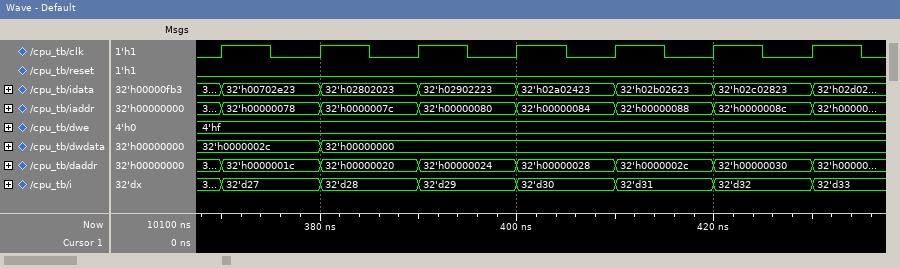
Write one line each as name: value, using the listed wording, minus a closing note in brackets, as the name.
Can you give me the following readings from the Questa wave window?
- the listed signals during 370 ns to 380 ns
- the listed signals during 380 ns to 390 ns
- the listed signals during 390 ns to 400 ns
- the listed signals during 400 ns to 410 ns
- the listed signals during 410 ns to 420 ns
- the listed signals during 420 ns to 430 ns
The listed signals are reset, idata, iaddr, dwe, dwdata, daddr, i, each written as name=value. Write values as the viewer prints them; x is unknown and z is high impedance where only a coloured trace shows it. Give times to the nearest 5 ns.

the listed signals during 370 ns to 380 ns: reset=0, idata=32'h00702e23, iaddr=32'h00000078, dwe=4'hf, dwdata=32'h0000002c, daddr=32'h0000001c, i=32'd27
the listed signals during 380 ns to 390 ns: reset=0, idata=32'h02802023, iaddr=32'h0000007c, dwe=4'hf, dwdata=32'h00000000, daddr=32'h00000020, i=32'd28
the listed signals during 390 ns to 400 ns: reset=0, idata=32'h02902223, iaddr=32'h00000080, dwe=4'hf, dwdata=32'h00000000, daddr=32'h00000024, i=32'd29
the listed signals during 400 ns to 410 ns: reset=0, idata=32'h02a02423, iaddr=32'h00000084, dwe=4'hf, dwdata=32'h00000000, daddr=32'h00000028, i=32'd30
the listed signals during 410 ns to 420 ns: reset=0, idata=32'h02b02623, iaddr=32'h00000088, dwe=4'hf, dwdata=32'h00000000, daddr=32'h0000002c, i=32'd31
the listed signals during 420 ns to 430 ns: reset=0, idata=32'h02c02823, iaddr=32'h0000008c, dwe=4'hf, dwdata=32'h00000000, daddr=32'h00000030, i=32'd32
